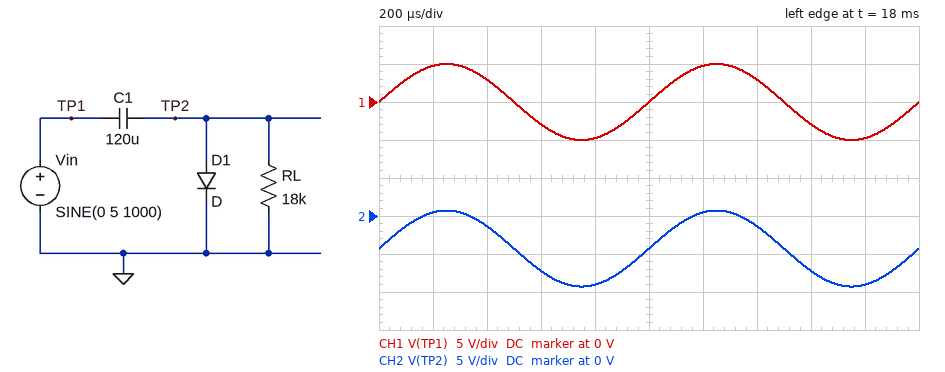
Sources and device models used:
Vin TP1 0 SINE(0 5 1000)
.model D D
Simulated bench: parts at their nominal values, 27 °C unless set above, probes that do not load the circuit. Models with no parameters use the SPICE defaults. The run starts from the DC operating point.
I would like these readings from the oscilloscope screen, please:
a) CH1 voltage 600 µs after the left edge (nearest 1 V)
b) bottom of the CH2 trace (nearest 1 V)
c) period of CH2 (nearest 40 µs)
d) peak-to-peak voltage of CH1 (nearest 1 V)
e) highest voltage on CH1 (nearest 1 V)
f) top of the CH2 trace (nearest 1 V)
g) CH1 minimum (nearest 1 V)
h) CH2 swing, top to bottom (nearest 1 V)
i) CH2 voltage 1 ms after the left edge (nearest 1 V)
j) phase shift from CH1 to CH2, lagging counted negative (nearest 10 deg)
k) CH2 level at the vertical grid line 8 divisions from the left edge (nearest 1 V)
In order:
-3 V
-9 V
1.00 ms
10 V
5 V
1 V
-5 V
10 V
-4 V
0 deg
-7 V
